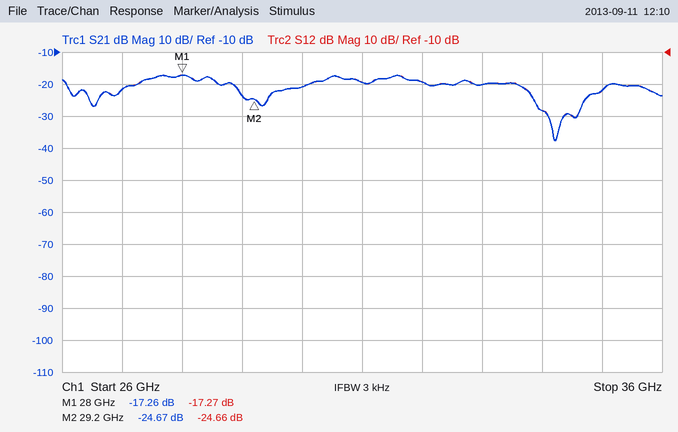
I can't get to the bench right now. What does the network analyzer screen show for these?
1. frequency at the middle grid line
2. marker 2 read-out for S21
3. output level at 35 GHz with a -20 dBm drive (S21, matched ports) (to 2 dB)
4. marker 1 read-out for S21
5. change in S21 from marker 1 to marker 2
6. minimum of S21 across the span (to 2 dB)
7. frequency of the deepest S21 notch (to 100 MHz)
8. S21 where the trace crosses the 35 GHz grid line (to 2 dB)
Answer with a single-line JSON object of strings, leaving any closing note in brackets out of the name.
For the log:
{"frequency at the middle grid line": "31 GHz", "marker 2 read-out for S21": "-24.67 dB", "output level at 35 GHz with a -20 dBm drive (S21, matched ports)": "-42 dBm", "marker 1 read-out for S21": "-17.26 dB", "change in S21 from marker 1 to marker 2": "-7.41 dB", "minimum of S21 across the span": "-38 dB", "frequency of the deepest S21 notch": "34.2 GHz", "S21 where the trace crosses the 35 GHz grid line": "-22 dB"}
